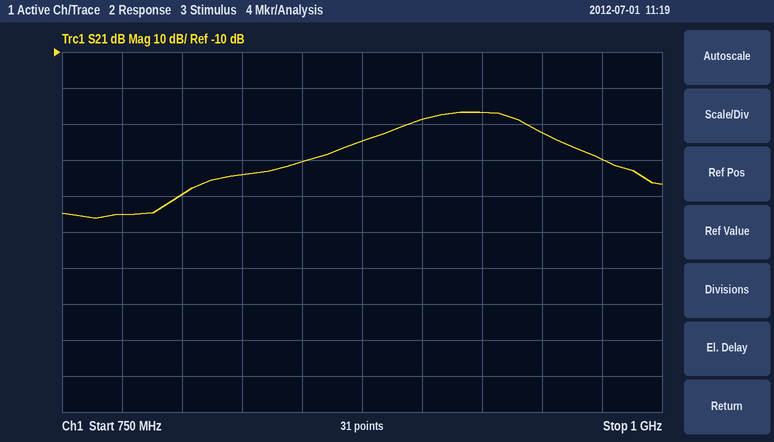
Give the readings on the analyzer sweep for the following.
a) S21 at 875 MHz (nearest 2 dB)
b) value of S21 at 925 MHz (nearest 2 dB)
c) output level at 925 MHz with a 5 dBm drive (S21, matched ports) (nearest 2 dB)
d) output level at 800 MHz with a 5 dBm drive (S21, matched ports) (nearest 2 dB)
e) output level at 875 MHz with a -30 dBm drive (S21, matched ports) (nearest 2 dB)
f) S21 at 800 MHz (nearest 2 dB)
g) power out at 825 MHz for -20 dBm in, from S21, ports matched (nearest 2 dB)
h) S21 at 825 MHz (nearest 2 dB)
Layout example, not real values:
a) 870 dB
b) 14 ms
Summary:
a) -34 dB
b) -26 dB
c) -22 dBm
d) -44 dBm
e) -64 dBm
f) -50 dB
g) -64 dBm
h) -44 dB
